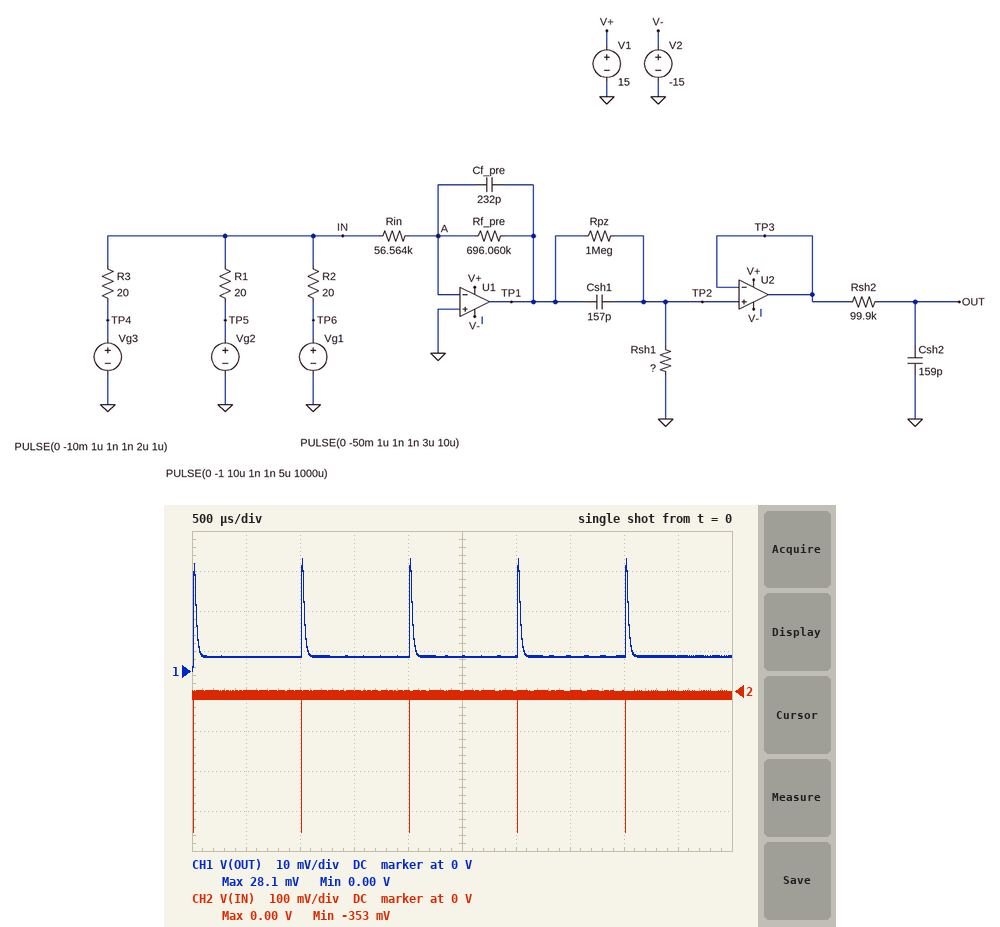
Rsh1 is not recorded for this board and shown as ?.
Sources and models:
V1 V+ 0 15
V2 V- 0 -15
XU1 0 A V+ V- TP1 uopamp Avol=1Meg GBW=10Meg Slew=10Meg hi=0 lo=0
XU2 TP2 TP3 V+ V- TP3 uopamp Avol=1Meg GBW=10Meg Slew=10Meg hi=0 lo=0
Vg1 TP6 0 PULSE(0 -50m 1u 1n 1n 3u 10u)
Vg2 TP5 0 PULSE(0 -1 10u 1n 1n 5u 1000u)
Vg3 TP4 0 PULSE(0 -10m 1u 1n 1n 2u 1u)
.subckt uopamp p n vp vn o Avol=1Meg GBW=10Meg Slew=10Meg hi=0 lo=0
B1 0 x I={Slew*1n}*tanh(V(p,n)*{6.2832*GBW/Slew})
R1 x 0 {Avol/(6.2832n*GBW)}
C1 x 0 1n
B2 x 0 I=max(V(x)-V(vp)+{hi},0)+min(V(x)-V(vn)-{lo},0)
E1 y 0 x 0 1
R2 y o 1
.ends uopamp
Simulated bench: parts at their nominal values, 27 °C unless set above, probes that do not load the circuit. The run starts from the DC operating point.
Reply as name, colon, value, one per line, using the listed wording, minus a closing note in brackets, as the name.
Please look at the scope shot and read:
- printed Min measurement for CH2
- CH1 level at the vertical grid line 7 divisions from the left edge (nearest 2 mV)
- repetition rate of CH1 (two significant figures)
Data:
printed Min measurement for CH2: -353 mV
CH1 level at the vertical grid line 7 divisions from the left edge: 4 mV
repetition rate of CH1: 1.0 kHz
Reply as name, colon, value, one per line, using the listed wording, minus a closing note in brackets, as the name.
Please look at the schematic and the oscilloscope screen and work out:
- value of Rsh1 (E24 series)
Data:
value of Rsh1: 36 kΩ
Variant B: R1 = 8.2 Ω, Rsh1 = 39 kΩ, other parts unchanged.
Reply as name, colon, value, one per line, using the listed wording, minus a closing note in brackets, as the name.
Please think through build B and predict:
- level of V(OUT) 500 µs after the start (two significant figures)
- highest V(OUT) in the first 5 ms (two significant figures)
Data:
level of V(OUT) 500 µs after the start: 2.6 mV
highest V(OUT) in the first 5 ms: 45 mV
